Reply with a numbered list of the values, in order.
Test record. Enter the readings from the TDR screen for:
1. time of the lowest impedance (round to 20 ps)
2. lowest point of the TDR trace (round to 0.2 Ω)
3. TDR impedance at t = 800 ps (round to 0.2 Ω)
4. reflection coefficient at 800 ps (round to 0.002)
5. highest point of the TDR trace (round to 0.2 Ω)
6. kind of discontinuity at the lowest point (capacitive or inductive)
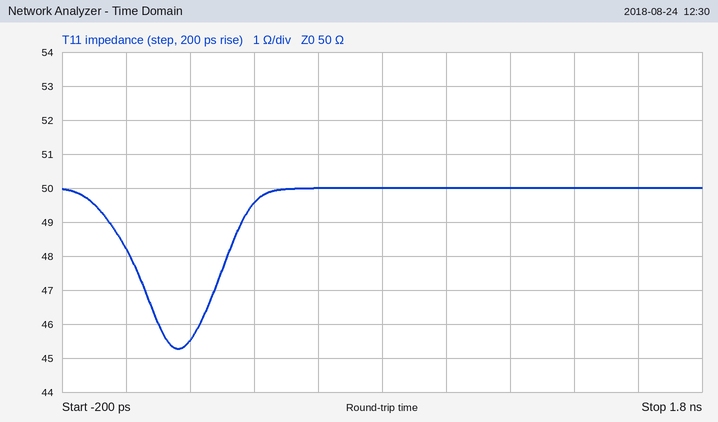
1. 160 ps
2. 45.2 Ω
3. 50.0 Ω
4. 0.000
5. 50.0 Ω
6. capacitive
